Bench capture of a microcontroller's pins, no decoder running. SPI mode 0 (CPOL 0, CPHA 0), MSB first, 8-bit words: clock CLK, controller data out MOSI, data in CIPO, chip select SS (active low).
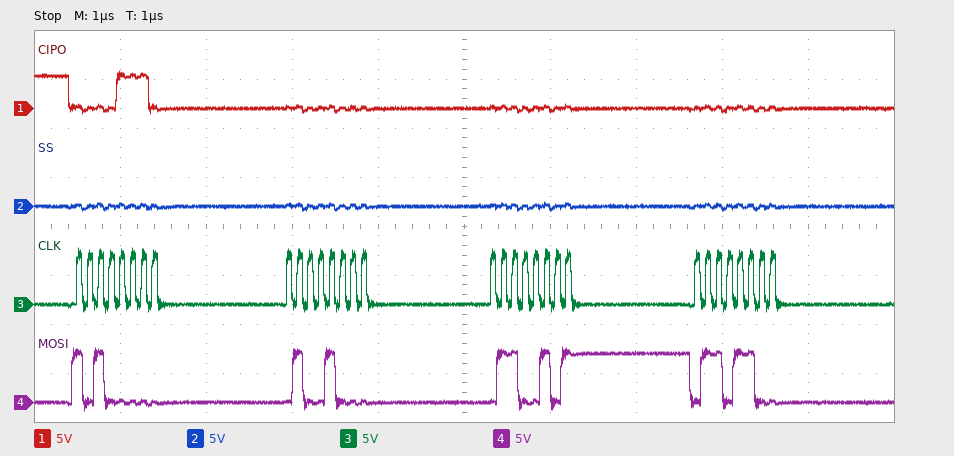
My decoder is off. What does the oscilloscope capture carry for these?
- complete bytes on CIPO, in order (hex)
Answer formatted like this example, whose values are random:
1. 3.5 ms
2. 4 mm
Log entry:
1. 0E 00 00 00
